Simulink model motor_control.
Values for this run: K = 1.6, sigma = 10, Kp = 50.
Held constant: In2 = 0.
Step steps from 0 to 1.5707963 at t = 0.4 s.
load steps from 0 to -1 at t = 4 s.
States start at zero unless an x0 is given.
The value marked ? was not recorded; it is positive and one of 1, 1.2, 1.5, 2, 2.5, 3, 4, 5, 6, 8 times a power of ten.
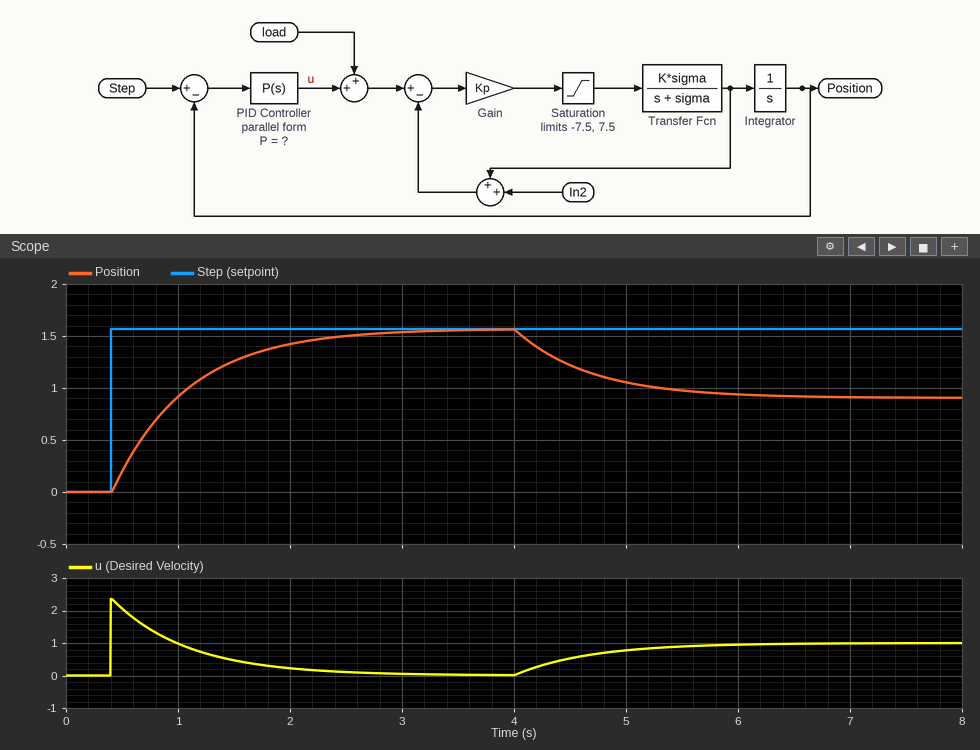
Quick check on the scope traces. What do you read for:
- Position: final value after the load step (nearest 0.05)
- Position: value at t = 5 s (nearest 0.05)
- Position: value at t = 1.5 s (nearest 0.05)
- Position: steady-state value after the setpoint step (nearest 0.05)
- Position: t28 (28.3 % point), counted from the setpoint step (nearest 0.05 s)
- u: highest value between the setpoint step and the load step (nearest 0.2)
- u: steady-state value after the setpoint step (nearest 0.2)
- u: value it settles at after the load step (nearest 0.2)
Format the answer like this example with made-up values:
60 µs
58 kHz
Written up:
0.90
1.05
1.25
1.55
0.25 s
2.4
0.0
1.0
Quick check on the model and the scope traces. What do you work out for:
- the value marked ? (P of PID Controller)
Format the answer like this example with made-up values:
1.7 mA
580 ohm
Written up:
1.5
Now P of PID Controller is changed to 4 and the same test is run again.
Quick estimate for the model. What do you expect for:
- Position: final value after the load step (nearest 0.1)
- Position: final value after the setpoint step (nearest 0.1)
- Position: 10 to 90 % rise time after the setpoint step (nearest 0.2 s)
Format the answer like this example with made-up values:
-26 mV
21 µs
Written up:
1.3
1.6
0.6 s
